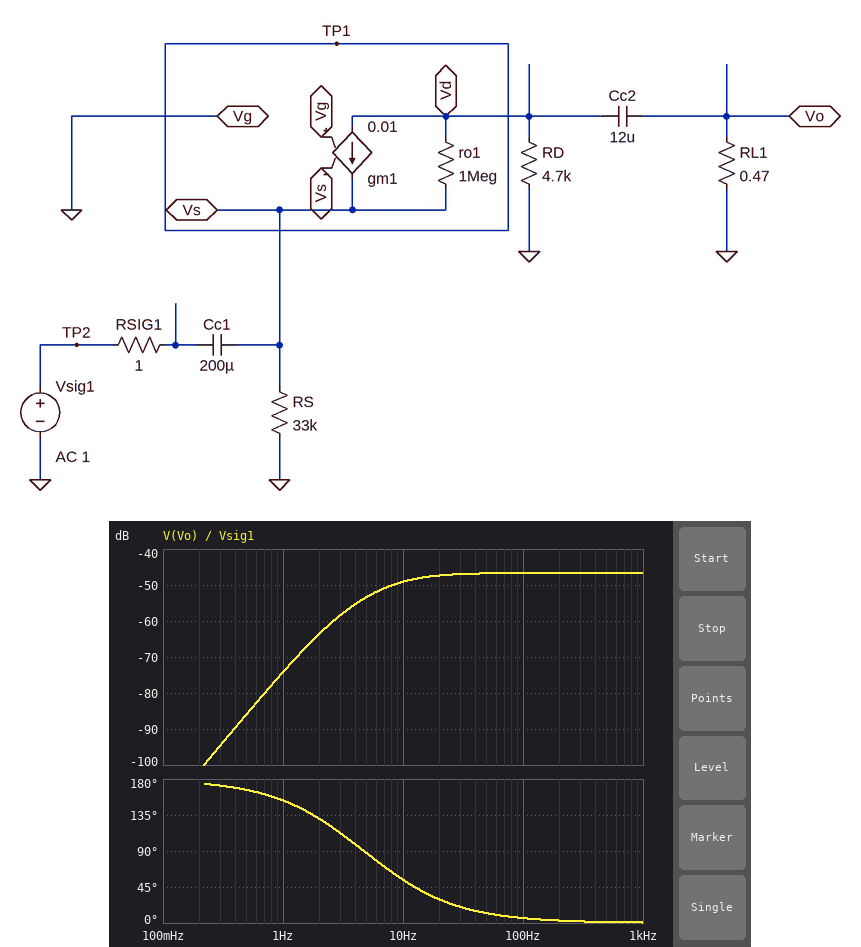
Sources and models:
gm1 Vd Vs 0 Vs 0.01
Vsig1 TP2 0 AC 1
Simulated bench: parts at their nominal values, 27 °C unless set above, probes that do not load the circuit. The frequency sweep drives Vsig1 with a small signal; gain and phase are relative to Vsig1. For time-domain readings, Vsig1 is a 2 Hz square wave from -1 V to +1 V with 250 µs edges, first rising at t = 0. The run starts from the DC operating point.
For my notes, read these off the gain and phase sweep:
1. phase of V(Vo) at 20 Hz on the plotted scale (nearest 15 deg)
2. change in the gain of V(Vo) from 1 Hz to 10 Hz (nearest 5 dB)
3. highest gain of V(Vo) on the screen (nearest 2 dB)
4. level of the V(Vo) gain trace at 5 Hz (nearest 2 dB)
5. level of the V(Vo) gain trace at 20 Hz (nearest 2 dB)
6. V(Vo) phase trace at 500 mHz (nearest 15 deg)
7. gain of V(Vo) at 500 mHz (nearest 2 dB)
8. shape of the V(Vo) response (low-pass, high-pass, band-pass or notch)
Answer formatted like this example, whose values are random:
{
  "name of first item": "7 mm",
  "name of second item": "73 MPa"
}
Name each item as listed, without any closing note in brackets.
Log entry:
{
  "phase of V(Vo) at 20 Hz on the plotted scale": "30 deg",
  "change in the gain of V(Vo) from 1 Hz to 10 Hz": "25 dB",
  "highest gain of V(Vo) on the screen": "-46 dB",
  "level of the V(Vo) gain trace at 5 Hz": "-54 dB",
  "level of the V(Vo) gain trace at 20 Hz": "-48 dB",
  "V(Vo) phase trace at 500 mHz": "165 deg",
  "gain of V(Vo) at 500 mHz": "-86 dB",
  "shape of the V(Vo) response": "high-pass"
}
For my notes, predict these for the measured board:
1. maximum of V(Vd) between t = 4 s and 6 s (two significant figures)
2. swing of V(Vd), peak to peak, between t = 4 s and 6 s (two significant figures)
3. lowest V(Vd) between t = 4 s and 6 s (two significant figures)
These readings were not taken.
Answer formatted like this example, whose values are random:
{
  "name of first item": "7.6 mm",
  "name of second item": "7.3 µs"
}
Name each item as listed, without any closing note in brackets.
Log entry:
{
  "maximum of V(Vd) between t = 4 s and 6 s": "18 V",
  "swing of V(Vd), peak to peak, between t = 4 s and 6 s": "37 V",
  "lowest V(Vd) between t = 4 s and 6 s": "-18 V"
}
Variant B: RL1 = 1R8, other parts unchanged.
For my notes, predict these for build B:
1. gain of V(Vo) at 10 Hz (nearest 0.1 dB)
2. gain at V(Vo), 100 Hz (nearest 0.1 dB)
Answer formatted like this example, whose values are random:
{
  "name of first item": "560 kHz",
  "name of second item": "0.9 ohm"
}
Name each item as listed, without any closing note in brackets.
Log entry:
{
  "gain of V(Vo) at 10 Hz": "-37.4 dB",
  "gain at V(Vo), 100 Hz": "-35.0 dB"
}
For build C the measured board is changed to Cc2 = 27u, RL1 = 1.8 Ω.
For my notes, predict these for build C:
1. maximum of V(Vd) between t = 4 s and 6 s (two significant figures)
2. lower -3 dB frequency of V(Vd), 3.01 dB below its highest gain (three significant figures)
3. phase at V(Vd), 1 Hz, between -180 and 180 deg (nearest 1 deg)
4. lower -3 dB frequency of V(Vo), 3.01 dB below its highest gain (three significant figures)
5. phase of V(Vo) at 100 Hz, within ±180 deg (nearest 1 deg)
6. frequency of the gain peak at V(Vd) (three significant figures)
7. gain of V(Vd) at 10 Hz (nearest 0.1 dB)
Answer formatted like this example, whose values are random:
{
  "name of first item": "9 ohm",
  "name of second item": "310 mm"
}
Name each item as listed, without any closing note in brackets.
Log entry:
{
  "maximum of V(Vd) between t = 4 s and 6 s": "8.9 V",
  "lower -3 dB frequency of V(Vd), 3.01 dB below its highest gain": "977 mHz",
  "phase at V(Vd), 1 Hz, between -180 and 180 deg": "44 deg",
  "lower -3 dB frequency of V(Vo), 3.01 dB below its highest gain": "8.10 Hz",
  "phase of V(Vo) at 100 Hz, within ±180 deg": "5 deg",
  "frequency of the gain peak at V(Vd)": "3.15 Hz",
  "gain of V(Vd) at 10 Hz": "13.1 dB"
}
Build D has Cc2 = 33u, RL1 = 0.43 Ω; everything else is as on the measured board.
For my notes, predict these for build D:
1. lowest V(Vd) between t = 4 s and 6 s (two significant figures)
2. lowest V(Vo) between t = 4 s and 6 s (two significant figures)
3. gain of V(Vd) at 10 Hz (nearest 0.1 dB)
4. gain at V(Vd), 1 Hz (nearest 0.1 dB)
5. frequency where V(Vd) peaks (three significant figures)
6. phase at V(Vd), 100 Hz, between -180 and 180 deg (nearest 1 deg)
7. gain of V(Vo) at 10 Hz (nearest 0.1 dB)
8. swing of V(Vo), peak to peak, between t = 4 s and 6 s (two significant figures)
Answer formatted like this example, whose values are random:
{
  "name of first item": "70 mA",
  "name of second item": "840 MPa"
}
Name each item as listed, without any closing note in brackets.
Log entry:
{
  "lowest V(Vd) between t = 4 s and 6 s": "-7.2 V",
  "lowest V(Vo) between t = 4 s and 6 s": "-8.7 mV",
  "gain of V(Vd) at 10 Hz": "11.4 dB",
  "gain at V(Vd), 1 Hz": "12.4 dB",
  "frequency where V(Vd) peaks": "2.85 Hz",
  "phase at V(Vd), 100 Hz, between -180 and 180 deg": "-84 deg",
  "gain of V(Vo) at 10 Hz": "-49.6 dB",
  "swing of V(Vo), peak to peak, between t = 4 s and 6 s": "17 mV"
}
